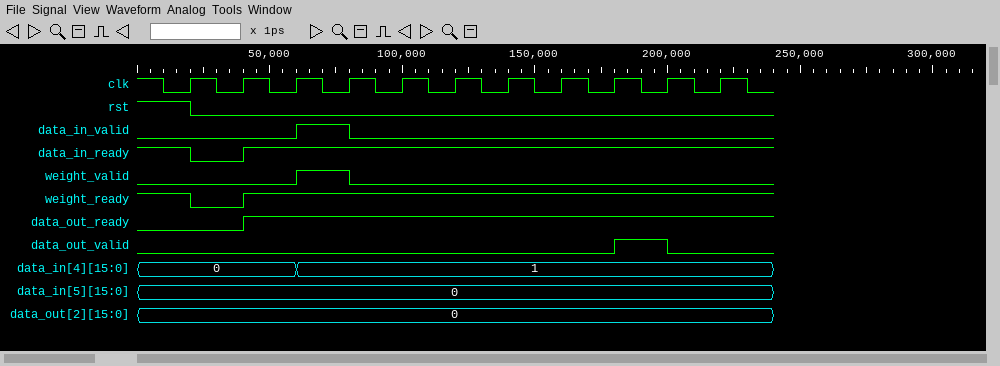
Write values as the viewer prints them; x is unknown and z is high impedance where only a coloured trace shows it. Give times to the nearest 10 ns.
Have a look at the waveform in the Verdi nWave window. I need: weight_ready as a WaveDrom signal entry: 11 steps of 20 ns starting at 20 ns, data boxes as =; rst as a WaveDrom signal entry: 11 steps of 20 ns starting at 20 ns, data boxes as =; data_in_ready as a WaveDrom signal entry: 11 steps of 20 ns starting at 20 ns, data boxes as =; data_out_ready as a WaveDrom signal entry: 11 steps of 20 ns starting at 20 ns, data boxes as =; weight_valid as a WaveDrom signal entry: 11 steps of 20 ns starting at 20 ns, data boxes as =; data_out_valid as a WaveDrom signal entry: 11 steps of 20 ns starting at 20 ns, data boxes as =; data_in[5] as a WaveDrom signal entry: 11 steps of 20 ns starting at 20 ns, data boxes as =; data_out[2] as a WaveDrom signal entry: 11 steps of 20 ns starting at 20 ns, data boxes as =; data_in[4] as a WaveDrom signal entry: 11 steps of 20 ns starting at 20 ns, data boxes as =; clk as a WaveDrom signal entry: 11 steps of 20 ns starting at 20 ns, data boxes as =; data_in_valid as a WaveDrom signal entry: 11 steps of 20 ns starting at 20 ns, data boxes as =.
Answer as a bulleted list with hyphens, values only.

- {name: 'weight_ready', wave: '01.........'}
- {name: 'rst', wave: '0..........'}
- {name: 'data_in_ready', wave: '01.........'}
- {name: 'data_out_ready', wave: '01.........'}
- {name: 'weight_valid', wave: '0.10.......'}
- {name: 'data_out_valid', wave: '0.......10.'}
- {name: 'data_in[5]', wave: '=..........', data: '0'}
- {name: 'data_out[2]', wave: '=..........', data: '0'}
- {name: 'data_in[4]', wave: '=.=........', data: '0 1'}
- {name: 'clk', wave: 'p..........'}
- {name: 'data_in_valid', wave: '0.10.......'}
